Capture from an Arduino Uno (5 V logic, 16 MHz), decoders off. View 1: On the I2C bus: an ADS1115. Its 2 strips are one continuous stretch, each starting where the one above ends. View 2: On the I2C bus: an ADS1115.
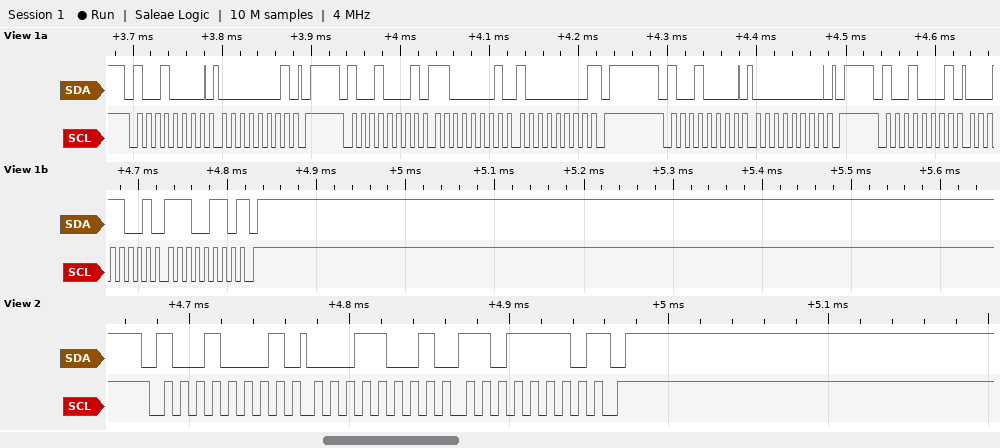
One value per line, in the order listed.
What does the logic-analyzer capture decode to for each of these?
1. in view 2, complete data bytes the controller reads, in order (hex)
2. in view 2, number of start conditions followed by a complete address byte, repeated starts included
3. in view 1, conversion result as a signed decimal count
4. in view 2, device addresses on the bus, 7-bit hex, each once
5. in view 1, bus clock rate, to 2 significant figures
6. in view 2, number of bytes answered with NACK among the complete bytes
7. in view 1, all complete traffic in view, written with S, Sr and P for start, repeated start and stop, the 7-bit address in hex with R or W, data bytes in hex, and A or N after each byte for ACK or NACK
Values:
19 DE
1
6630
0x48
100 kHz
1
S 48W A 01 A P S 48R A C1 A 80 N P S 48W A 00 A P S 48R A 19 A E6 N P
